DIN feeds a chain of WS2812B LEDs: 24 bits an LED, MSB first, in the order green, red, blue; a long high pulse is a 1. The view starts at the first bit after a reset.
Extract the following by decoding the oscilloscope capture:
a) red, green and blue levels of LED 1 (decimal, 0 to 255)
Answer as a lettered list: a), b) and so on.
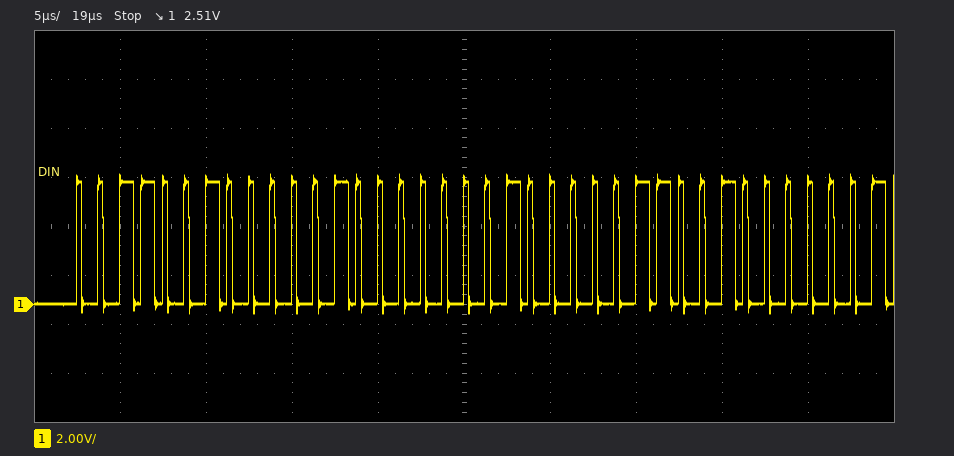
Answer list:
a) 8, 50, 8
